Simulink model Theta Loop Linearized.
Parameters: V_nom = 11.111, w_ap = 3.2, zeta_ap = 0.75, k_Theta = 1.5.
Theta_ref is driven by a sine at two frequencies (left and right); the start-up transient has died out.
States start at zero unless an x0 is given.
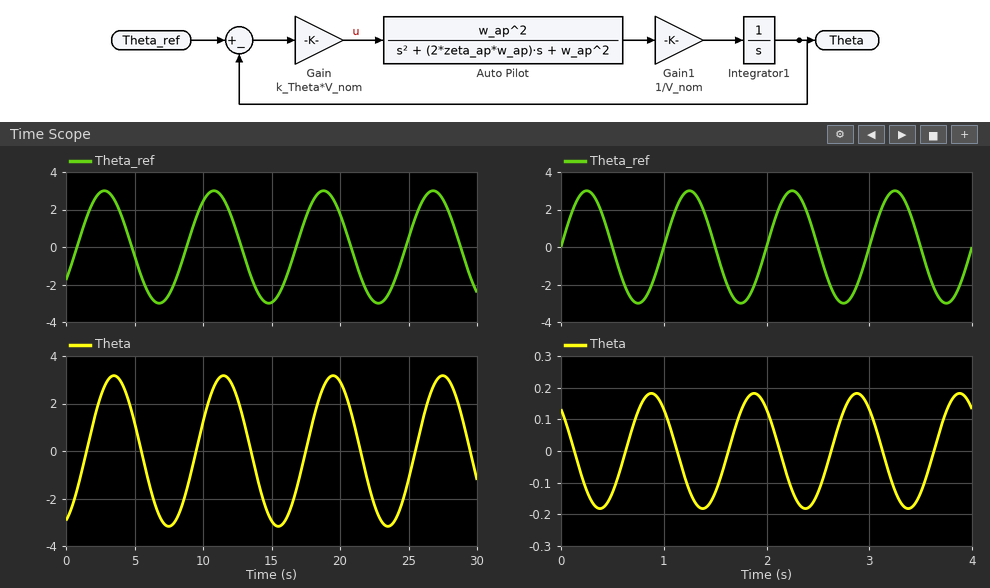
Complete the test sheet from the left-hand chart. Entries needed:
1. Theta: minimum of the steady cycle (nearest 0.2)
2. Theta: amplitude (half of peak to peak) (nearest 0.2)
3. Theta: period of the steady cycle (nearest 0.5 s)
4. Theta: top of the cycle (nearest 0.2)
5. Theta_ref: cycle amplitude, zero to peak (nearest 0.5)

-3.2
3.2
8.0 s
3.2
3.0
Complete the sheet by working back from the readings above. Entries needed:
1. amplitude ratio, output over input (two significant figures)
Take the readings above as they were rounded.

1.1
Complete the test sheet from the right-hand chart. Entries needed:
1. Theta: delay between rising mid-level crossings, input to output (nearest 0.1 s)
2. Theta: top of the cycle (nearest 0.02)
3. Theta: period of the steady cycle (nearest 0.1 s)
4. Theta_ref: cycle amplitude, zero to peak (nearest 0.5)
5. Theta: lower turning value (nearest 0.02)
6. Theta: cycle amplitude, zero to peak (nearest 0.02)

0.6 s
0.18
1.0 s
3.0
-0.18
0.18
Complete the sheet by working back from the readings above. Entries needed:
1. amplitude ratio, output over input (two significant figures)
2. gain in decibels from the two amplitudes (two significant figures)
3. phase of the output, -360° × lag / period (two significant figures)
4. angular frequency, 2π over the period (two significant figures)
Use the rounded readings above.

0.060
-24 dB
-220°
6.3 rad/s
